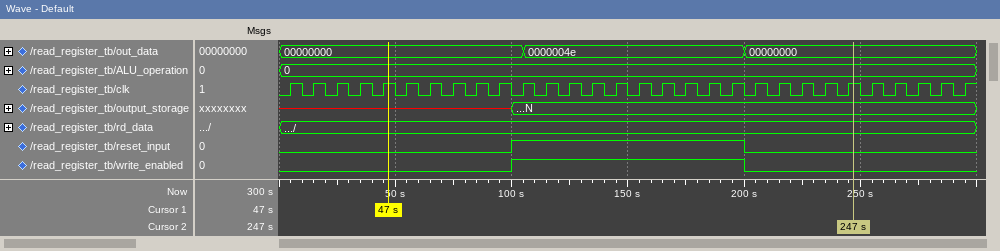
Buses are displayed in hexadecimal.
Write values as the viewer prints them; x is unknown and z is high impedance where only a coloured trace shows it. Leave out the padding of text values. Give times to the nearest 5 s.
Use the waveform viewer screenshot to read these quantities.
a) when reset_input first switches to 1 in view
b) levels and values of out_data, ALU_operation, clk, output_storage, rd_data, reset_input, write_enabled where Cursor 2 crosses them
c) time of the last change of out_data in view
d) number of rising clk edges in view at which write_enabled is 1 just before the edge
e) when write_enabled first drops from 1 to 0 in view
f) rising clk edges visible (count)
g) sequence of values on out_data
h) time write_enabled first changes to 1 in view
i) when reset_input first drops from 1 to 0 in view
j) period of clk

100 s
out_data=00000000, ALU_operation=0, clk=1, output_storage=N, rd_data=/, reset_input=0, write_enabled=0
200 s
10
200 s
30
00000000, 0000004e, 00000000
100 s
200 s
10 s
